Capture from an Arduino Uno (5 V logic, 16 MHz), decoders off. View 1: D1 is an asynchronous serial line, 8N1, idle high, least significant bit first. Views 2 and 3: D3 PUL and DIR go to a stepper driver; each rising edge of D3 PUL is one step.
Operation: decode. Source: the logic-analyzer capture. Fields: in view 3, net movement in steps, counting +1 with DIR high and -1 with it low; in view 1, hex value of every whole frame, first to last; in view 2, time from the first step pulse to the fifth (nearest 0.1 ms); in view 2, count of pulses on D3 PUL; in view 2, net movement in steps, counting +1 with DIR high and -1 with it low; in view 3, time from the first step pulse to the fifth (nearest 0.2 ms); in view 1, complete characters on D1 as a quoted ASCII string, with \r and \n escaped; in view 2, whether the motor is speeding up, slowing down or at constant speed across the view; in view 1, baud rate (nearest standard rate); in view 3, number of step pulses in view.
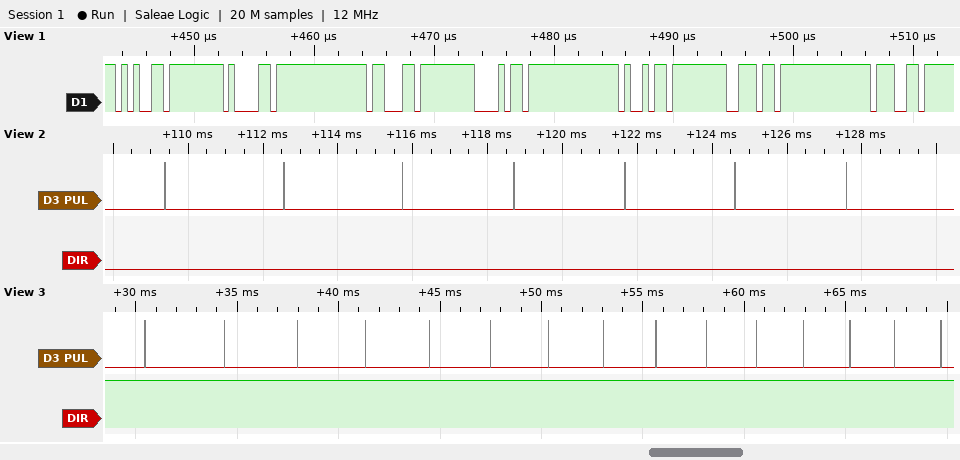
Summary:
+15
65 61 63 68 69 6E 67
12.3 ms
7
-7
14.0 ms
"eaching"
speeding up
2000000 baud
15
